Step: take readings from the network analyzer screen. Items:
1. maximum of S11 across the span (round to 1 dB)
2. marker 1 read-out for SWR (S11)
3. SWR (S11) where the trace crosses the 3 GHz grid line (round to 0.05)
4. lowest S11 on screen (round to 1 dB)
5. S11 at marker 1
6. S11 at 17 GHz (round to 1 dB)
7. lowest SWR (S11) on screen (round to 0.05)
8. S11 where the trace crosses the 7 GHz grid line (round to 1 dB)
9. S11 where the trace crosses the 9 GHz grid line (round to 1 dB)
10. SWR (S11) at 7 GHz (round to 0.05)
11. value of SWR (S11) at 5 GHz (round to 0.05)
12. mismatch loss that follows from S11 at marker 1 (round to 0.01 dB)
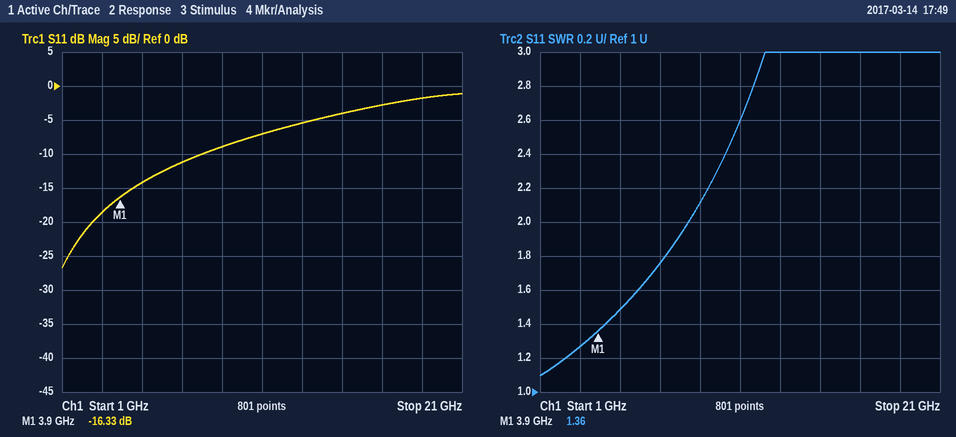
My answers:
-1 dB
1.36
1.25
-27 dB
-16.33 dB
-3 dB
1.10
-11 dB
-9 dB
1.75
1.50
0.10 dB
